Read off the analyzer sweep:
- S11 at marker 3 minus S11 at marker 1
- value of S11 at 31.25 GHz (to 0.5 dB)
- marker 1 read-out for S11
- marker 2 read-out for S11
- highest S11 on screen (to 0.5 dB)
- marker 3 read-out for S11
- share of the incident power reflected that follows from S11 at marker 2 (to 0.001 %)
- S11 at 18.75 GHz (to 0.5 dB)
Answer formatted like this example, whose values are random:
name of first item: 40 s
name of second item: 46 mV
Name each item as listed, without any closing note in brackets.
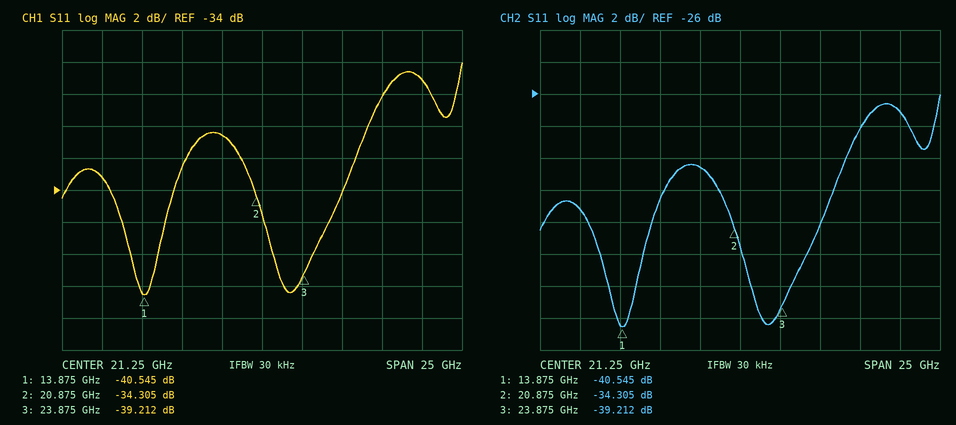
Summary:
S11 at marker 3 minus S11 at marker 1: 1.333 dB
value of S11 at 31.25 GHz: -27.0 dB
marker 1 read-out for S11: -40.545 dB
marker 2 read-out for S11: -34.305 dB
highest S11 on screen: -26.0 dB
marker 3 read-out for S11: -39.212 dB
share of the incident power reflected that follows from S11 at marker 2: 0.037 %
S11 at 18.75 GHz: -30.5 dB
